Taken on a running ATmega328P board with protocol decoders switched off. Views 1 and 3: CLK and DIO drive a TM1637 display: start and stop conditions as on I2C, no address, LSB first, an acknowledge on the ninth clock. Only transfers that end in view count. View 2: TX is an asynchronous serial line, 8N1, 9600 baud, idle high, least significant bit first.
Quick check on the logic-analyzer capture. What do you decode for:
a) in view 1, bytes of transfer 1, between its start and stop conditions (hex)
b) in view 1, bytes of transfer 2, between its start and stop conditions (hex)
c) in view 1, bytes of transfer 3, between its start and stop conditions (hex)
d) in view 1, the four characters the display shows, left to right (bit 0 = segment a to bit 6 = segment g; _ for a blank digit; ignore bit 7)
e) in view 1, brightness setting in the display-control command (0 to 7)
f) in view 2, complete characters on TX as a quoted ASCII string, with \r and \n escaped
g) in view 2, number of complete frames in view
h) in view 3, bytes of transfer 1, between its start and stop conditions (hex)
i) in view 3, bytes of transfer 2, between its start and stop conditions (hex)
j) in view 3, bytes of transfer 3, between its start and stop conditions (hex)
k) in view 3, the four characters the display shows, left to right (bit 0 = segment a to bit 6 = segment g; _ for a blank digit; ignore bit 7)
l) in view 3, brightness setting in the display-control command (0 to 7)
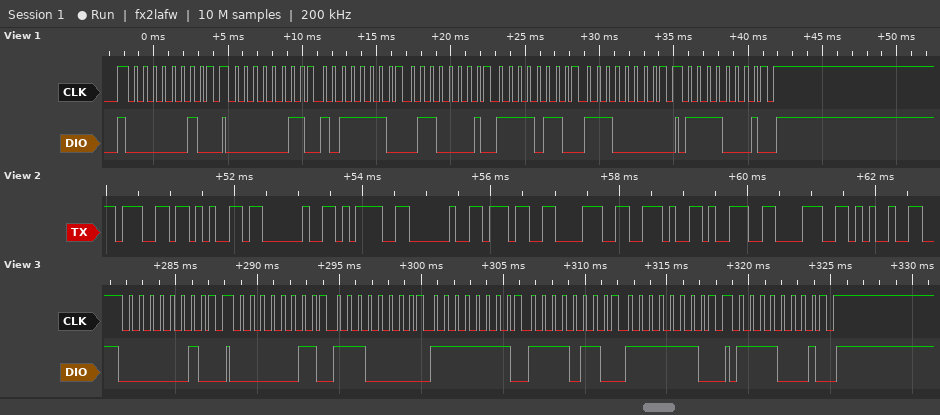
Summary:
40
C0 7D 86 6F 07
8F
6197
7
"ge = 78.98%"
11
40
C0 07 FF 6F 7F
8F
7898
7
